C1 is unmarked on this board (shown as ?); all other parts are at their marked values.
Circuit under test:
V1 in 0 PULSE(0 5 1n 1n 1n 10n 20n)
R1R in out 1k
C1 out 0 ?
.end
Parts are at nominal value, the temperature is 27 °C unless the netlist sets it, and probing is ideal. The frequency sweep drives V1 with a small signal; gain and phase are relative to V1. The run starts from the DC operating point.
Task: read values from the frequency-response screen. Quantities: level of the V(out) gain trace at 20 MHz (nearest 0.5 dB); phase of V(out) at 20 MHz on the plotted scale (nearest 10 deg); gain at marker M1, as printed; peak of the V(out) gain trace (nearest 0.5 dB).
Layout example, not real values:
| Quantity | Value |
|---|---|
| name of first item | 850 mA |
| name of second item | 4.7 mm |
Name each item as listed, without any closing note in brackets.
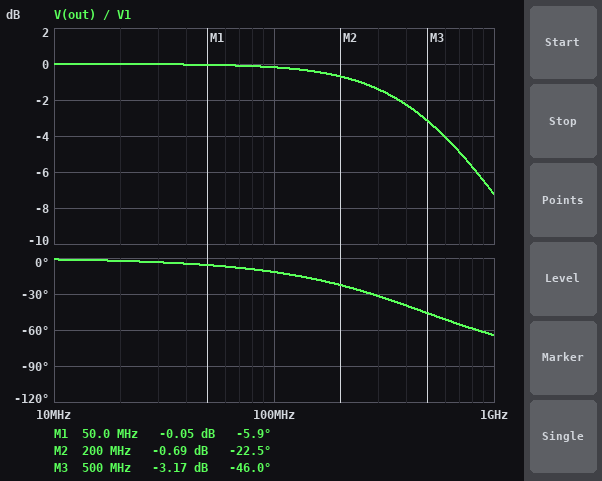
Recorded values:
| Quantity | Value |
|---|---|
| level of the V(out) gain trace at 20 MHz | 0 dB |
| phase of V(out) at 20 MHz on the plotted scale | 0 deg |
| gain at marker M1, as printed | -0.05 dB |
| peak of the V(out) gain trace | 0 dB |
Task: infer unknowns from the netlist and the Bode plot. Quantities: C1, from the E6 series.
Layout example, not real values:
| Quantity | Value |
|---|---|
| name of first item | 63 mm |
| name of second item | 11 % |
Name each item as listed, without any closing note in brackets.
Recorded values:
| Quantity | Value |
|---|---|
| C1, from the E6 series | 330 fF |
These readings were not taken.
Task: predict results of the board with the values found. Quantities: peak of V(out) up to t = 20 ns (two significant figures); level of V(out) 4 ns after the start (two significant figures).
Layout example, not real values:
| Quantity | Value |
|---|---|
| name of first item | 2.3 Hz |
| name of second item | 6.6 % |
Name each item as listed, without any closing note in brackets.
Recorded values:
| Quantity | Value |
|---|---|
| peak of V(out) up to t = 20 ns | 5.0 V |
| level of V(out) 4 ns after the start | 5.0 V |
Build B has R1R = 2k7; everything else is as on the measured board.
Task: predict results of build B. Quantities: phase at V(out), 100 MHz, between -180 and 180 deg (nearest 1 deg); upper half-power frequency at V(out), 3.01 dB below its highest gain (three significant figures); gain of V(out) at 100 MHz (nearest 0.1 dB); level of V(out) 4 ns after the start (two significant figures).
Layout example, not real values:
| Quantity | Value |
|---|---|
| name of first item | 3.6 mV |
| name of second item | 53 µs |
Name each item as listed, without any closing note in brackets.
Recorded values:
| Quantity | Value |
|---|---|
| phase at V(out), 100 MHz, between -180 and 180 deg | -29 deg |
| upper half-power frequency at V(out), 3.01 dB below its highest gain | 179 MHz |
| gain of V(out) at 100 MHz | -1.2 dB |
| level of V(out) 4 ns after the start | 4.7 V |
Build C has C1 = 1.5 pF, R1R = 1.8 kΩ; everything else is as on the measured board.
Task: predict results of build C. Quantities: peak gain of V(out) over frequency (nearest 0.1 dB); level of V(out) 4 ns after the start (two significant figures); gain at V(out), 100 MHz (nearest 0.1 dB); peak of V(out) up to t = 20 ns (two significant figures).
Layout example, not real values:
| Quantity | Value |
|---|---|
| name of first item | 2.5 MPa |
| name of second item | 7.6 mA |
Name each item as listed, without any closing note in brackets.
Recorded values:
| Quantity | Value |
|---|---|
| peak gain of V(out) over frequency | 0 dB |
| level of V(out) 4 ns after the start | 3.0 V |
| gain at V(out), 100 MHz | -5.9 dB |
| peak of V(out) up to t = 20 ns | 4.9 V |
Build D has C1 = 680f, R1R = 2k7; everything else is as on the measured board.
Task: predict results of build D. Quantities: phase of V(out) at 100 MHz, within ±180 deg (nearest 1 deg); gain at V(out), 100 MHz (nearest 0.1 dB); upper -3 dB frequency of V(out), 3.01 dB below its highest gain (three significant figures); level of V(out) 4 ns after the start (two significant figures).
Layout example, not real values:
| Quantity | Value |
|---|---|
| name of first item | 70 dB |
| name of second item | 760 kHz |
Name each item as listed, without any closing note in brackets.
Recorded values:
| Quantity | Value |
|---|---|
| phase of V(out) at 100 MHz, within ±180 deg | -49 deg |
| gain at V(out), 100 MHz | -3.7 dB |
| upper -3 dB frequency of V(out), 3.01 dB below its highest gain | 86.7 MHz |
| level of V(out) 4 ns after the start | 3.7 V |
